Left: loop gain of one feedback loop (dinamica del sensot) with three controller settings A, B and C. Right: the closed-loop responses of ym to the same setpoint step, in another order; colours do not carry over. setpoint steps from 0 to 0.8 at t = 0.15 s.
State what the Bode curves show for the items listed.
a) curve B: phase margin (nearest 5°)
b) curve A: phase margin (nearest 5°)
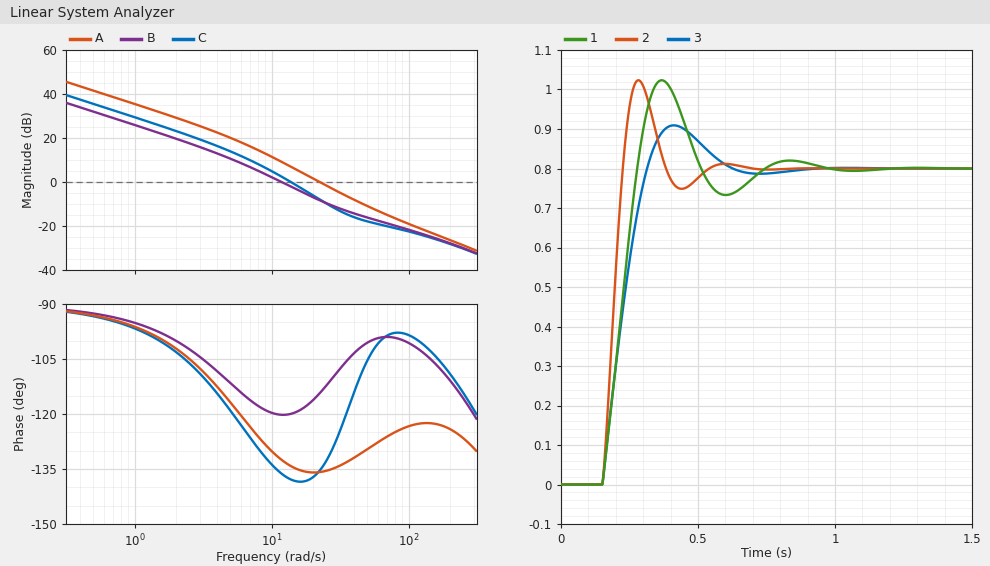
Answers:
60°
45°
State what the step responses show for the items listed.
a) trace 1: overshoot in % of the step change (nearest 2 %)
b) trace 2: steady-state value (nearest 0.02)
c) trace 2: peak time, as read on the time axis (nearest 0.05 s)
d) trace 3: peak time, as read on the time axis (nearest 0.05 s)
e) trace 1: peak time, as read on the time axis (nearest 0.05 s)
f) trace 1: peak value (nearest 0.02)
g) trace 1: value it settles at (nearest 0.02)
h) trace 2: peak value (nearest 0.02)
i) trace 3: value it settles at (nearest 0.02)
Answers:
28 %
0.80
0.30 s
0.40 s
0.35 s
1.02
0.80
1.02
0.80
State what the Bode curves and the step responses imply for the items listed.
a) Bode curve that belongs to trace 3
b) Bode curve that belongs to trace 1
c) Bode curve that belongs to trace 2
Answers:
B
C
A
